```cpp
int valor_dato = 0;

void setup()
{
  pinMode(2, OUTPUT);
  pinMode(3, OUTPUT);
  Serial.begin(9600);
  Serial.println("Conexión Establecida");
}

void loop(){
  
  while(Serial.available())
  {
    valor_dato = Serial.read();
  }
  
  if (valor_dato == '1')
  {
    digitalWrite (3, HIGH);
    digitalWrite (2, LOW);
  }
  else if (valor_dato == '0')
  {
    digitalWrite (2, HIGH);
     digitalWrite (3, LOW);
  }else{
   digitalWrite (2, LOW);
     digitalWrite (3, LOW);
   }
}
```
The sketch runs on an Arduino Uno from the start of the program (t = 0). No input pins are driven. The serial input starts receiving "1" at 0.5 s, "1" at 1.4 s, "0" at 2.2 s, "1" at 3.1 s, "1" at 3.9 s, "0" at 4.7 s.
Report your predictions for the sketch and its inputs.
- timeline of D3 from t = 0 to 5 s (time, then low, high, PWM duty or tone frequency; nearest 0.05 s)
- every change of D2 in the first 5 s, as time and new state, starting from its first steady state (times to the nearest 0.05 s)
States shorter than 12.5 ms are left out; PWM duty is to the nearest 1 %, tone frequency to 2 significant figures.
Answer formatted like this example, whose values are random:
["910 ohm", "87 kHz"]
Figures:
["0 s low; 0.5 s high; 2.2 s low; 3.1 s high; 4.7 s low", "0 s low; 2.2 s high; 3.1 s low; 4.7 s high"]
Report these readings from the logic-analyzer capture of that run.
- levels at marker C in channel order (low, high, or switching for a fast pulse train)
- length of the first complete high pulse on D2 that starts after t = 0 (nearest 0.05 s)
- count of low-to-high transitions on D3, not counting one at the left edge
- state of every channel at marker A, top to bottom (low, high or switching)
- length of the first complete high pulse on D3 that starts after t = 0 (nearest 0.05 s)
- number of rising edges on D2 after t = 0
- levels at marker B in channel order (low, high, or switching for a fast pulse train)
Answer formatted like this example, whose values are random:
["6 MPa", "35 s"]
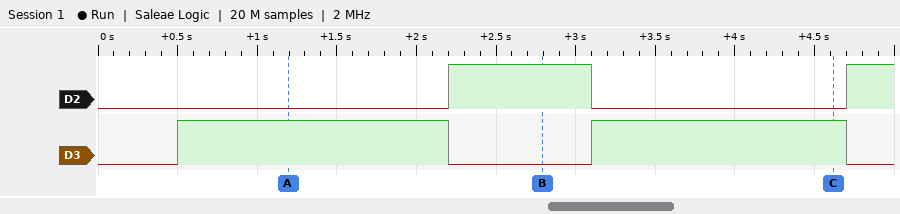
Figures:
["D2 low, D3 high", "0.90 s", "2", "D2 low, D3 high", "1.70 s", "2", "D2 high, D3 low"]
